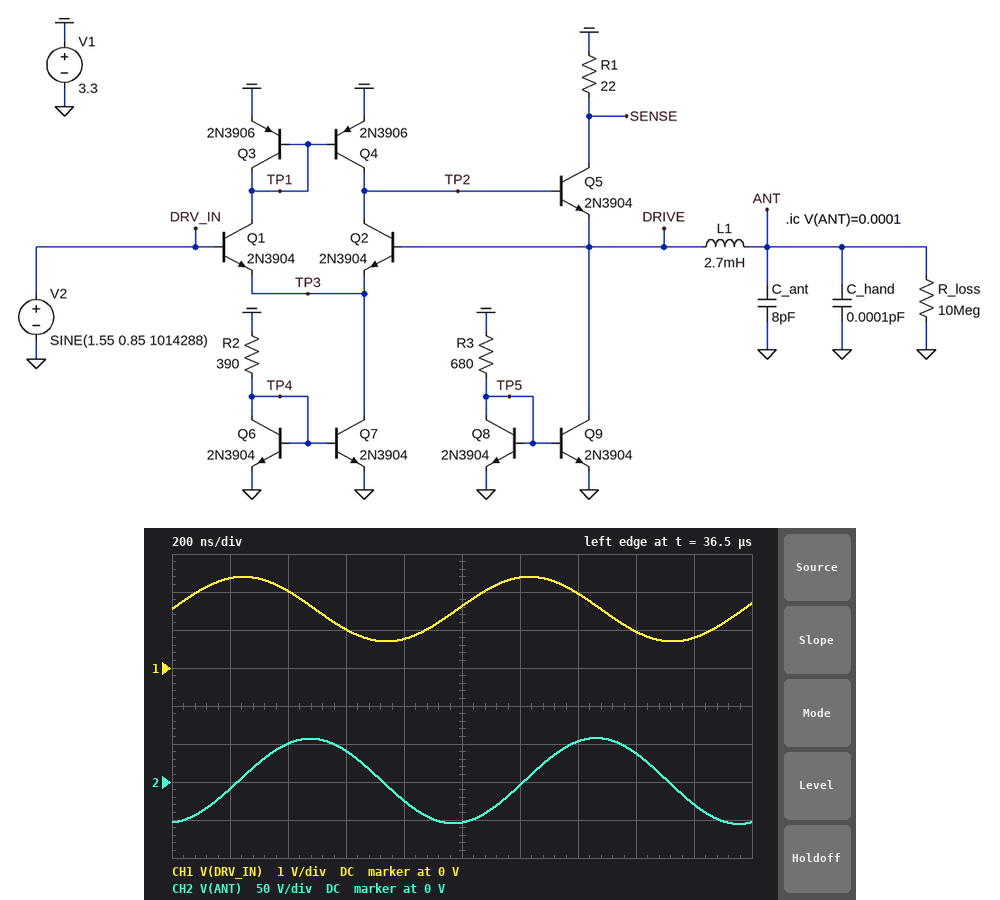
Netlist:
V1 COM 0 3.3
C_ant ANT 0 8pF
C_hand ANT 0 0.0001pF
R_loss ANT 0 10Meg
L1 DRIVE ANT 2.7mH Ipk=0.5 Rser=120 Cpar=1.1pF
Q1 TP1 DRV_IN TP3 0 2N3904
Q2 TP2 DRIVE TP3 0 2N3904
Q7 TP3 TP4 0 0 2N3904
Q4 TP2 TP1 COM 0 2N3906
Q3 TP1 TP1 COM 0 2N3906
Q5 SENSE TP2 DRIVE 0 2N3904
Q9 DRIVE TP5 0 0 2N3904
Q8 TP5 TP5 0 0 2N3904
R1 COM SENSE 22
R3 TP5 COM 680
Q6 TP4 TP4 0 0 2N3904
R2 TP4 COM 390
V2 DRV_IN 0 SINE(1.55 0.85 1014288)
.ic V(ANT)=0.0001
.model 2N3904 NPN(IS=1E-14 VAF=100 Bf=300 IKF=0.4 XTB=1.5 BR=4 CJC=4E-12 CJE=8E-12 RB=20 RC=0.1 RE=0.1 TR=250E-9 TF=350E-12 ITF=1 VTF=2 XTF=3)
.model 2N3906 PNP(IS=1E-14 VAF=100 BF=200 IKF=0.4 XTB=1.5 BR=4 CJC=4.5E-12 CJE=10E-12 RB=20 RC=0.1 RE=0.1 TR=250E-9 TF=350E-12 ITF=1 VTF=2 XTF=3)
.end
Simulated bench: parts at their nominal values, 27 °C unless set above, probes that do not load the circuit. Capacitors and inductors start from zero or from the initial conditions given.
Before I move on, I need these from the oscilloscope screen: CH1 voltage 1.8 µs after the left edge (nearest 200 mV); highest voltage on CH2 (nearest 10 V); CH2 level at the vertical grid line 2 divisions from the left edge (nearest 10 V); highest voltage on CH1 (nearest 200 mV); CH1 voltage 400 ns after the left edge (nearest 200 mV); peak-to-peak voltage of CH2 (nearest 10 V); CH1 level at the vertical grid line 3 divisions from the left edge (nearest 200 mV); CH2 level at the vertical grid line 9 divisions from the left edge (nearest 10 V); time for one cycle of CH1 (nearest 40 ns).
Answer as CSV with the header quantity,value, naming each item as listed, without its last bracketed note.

quantity,value
CH1 voltage 1.8 µs after the left edge,800 mV
highest voltage on CH2,60 V
CH2 level at the vertical grid line 2 divisions from the left edge,50 V
highest voltage on CH1,2.4 V
CH1 voltage 400 ns after the left edge,2.0 V
peak-to-peak voltage of CH2,110 V
CH1 level at the vertical grid line 3 divisions from the left edge,1.0 V
CH2 level at the vertical grid line 9 divisions from the left edge,-30 V
time for one cycle of CH1,1.00 µs
